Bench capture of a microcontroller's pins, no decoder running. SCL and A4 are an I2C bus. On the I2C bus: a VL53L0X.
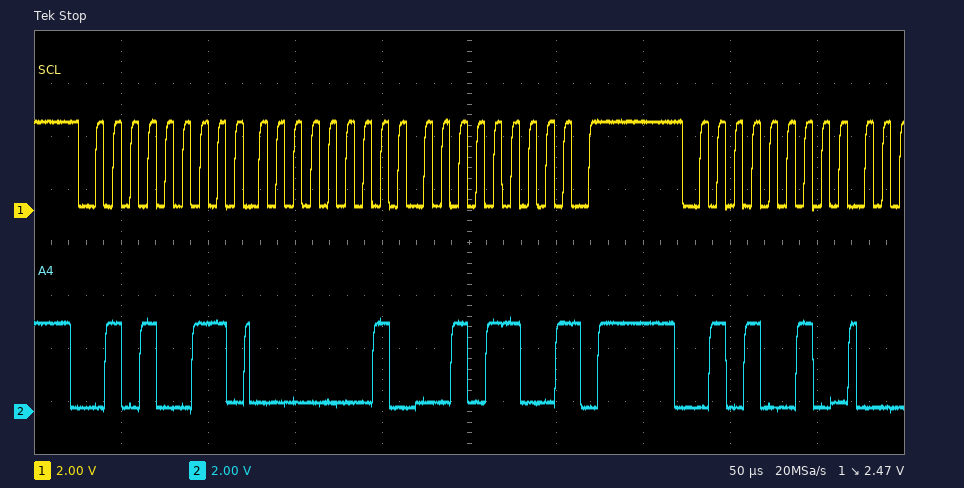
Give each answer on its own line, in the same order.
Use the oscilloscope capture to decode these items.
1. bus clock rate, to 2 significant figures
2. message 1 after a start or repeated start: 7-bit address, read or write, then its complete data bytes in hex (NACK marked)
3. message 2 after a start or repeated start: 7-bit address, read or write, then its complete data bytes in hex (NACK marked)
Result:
100 kHz
0x29 read: 01 2C NACK
0x29 write
